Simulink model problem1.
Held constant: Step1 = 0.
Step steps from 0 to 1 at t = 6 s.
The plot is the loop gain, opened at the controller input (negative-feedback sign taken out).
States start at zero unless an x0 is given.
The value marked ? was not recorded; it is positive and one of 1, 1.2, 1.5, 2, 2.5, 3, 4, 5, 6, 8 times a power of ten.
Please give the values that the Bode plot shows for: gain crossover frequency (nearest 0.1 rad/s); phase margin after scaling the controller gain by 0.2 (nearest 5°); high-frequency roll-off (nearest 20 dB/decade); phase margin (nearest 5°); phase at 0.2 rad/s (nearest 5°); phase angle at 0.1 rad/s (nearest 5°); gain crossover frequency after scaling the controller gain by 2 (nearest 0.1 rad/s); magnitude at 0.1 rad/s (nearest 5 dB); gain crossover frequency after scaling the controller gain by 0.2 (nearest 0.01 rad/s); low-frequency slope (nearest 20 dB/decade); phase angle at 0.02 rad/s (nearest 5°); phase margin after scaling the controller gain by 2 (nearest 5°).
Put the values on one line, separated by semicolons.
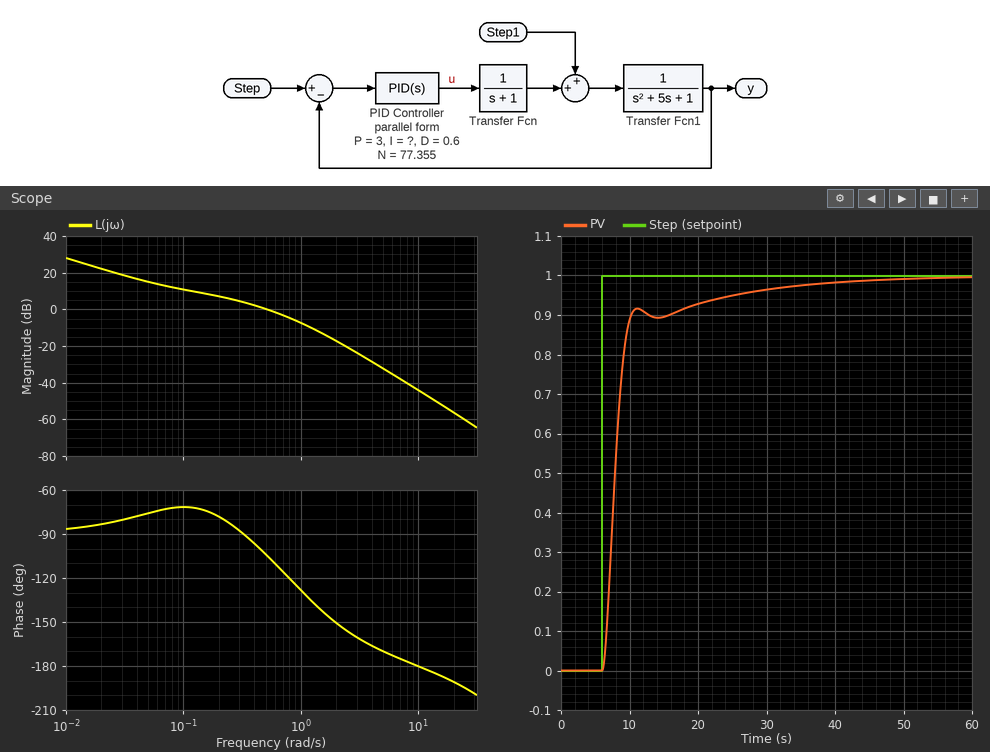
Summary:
0.5 rad/s; 105°; -40 dB/decade; 75°; -80°; -70°; 0.9 rad/s; 10 dB; 0.06 rad/s; -20 dB/decade; -85°; 55°
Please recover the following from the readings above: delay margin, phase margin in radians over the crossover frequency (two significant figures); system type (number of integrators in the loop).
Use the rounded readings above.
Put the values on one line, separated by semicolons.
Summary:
2.6 s; 1
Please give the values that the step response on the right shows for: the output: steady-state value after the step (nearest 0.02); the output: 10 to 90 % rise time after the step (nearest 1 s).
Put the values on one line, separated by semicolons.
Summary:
1.00; 4 s
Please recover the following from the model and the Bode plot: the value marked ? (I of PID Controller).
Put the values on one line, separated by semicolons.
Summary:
0.25
